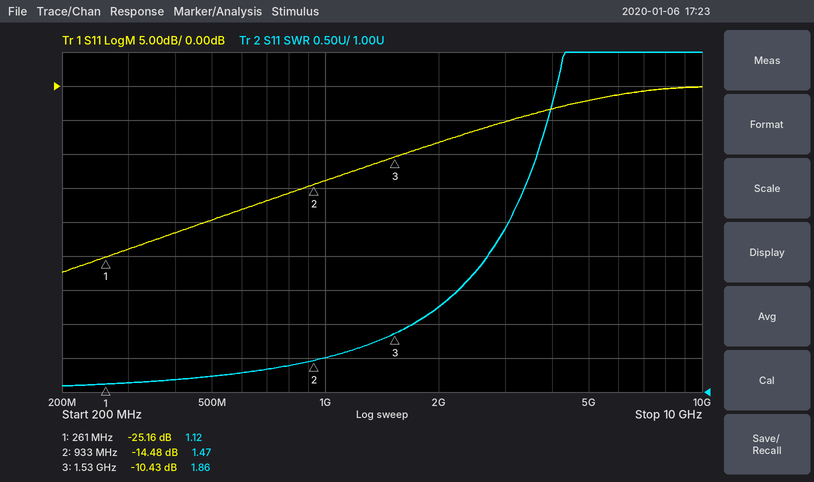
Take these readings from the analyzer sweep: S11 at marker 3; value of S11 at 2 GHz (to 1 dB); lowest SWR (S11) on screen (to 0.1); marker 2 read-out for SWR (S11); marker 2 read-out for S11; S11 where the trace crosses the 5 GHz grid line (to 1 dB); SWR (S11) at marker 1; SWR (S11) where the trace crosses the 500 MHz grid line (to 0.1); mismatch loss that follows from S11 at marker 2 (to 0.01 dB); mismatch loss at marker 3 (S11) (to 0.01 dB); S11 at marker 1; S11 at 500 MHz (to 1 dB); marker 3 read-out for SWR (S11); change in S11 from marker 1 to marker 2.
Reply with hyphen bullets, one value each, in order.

- -10.43 dB
- -8 dB
- 1.1
- 1.47
- -14.48 dB
- -2 dB
- 1.12
- 1.2
- 0.16 dB
- 0.41 dB
- -25.16 dB
- -20 dB
- 1.86
- 10.68 dB
